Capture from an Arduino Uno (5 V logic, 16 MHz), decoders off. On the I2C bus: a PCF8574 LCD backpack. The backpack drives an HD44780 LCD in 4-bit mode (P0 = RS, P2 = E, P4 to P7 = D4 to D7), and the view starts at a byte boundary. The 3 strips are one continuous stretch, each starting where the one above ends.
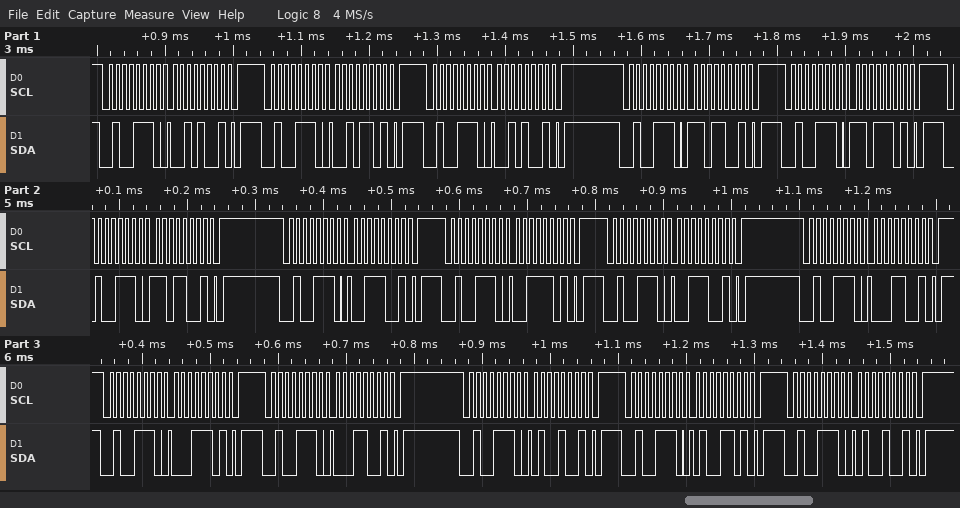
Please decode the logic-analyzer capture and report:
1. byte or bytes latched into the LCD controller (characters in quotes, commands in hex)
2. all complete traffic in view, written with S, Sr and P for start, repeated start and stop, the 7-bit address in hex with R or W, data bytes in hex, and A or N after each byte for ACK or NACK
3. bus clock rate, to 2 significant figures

'-' '1'
S 27W A 29 A P S 27W A 2D A P S 27W A 29 A P S 27W A D9 A P S 27W A DD A P S 27W A D9 A P S 27W A 39 A P S 27W A 3D A P S 27W A 39 A P S 27W A 19 A P S 27W A 1D A P S 27W A 19 A P S 27W A 49 A P S 27W A 4D A P S 27W A 49 A P
100 kHz
